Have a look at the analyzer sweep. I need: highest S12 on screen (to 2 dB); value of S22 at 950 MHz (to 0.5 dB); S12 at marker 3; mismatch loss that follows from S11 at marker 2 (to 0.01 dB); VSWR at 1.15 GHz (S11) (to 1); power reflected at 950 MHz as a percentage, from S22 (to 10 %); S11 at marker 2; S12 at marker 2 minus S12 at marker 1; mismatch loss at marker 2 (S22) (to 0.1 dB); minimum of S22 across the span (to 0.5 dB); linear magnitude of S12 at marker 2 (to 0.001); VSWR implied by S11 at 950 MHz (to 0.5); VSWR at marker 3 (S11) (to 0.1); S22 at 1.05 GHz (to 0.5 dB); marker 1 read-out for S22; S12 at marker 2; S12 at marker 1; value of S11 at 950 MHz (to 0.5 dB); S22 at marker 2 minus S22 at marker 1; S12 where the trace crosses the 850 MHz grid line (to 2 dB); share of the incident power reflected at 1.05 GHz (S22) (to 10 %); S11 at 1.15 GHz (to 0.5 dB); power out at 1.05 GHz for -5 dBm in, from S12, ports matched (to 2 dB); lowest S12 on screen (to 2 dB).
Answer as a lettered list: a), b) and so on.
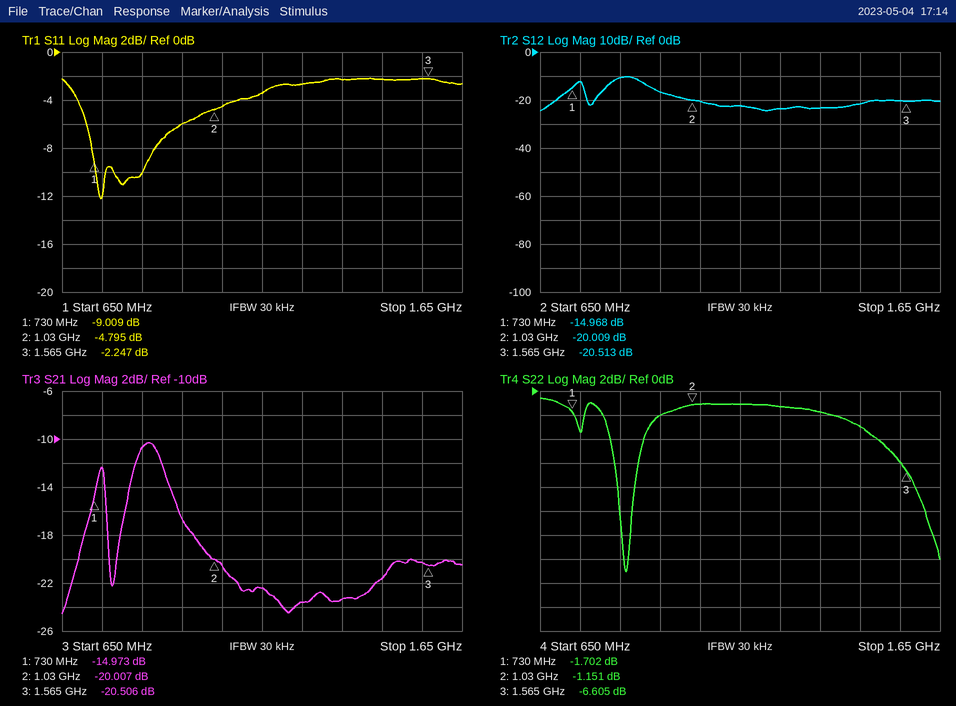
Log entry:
a) -10 dB
b) -2.0 dB
c) -20.513 dB
d) 1.75 dB
e) 5
f) 60 %
g) -4.795 dB
h) -5.041 dB
i) 6.3 dB
j) -15.0 dB
k) 0.100
l) 3.0
m) 7.8
n) -1.0 dB
o) -1.702 dB
p) -20.009 dB
q) -14.968 dB
r) -6.0 dB
s) 0.551 dB
t) -10 dB
u) 80 %
v) -3.5 dB
w) -26 dBm
x) -24 dB
